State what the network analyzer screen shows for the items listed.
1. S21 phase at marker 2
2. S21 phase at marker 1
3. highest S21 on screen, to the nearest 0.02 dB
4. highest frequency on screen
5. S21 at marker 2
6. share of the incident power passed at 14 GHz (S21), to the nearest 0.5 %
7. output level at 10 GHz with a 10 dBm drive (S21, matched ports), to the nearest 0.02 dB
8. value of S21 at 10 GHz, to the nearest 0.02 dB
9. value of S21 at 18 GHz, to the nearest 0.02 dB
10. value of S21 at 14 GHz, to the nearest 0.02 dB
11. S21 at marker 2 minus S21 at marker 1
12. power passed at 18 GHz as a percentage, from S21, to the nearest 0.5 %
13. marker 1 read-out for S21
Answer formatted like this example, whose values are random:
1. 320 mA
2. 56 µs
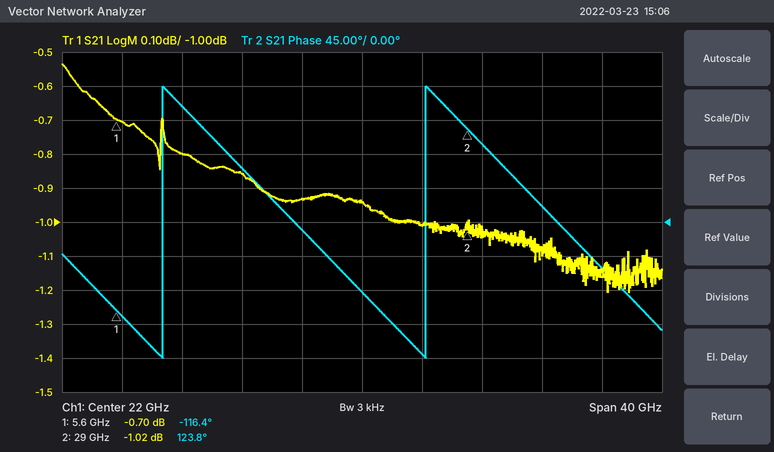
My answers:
1. 123.8°
2. -116.4°
3. -0.54 dB
4. 42 GHz
5. -1.02 dB
6. 82.0 %
7. 9.20 dBm
8. -0.80 dB
9. -0.94 dB
10. -0.86 dB
11. -0.32 dB
12. 80.5 %
13. -0.70 dB
